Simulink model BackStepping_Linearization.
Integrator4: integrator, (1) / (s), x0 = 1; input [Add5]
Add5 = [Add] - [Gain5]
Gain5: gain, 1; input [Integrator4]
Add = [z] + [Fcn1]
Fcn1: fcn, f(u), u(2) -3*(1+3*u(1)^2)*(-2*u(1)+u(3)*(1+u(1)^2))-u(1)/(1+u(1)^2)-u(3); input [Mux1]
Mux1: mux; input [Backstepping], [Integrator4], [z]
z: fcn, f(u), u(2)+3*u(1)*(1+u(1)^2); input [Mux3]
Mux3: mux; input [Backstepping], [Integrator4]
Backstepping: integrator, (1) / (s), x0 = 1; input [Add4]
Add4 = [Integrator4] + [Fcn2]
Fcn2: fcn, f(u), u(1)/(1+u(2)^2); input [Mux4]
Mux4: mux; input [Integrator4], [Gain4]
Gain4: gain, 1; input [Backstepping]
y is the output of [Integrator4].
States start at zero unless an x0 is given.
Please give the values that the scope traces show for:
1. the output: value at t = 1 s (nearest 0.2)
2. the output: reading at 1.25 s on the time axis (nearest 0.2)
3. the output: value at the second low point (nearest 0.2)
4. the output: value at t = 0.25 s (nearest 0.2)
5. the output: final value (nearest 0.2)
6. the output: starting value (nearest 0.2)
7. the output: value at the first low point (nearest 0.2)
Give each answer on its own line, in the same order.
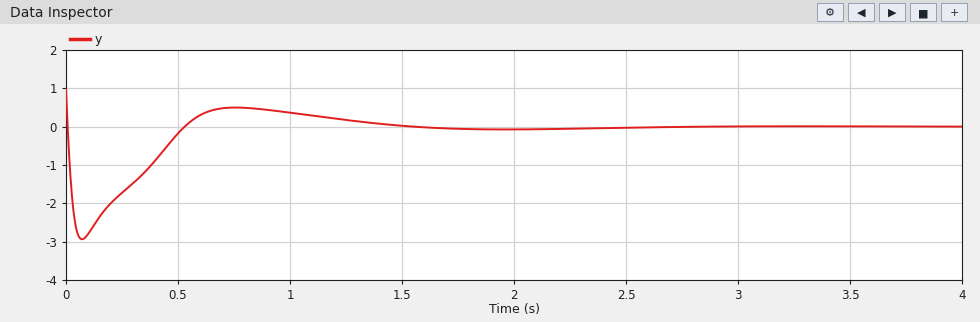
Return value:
0.4
0.2
0.0
-1.8
0.0
1.0
-3.0
